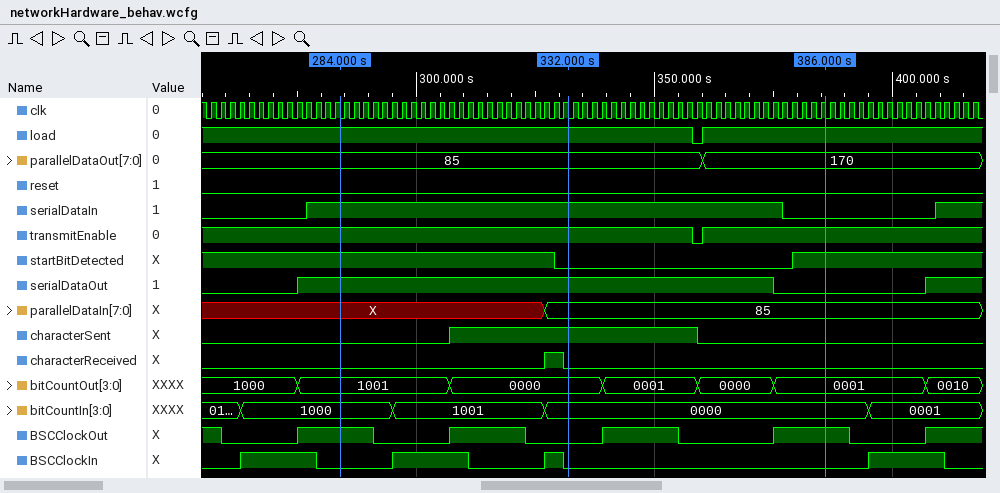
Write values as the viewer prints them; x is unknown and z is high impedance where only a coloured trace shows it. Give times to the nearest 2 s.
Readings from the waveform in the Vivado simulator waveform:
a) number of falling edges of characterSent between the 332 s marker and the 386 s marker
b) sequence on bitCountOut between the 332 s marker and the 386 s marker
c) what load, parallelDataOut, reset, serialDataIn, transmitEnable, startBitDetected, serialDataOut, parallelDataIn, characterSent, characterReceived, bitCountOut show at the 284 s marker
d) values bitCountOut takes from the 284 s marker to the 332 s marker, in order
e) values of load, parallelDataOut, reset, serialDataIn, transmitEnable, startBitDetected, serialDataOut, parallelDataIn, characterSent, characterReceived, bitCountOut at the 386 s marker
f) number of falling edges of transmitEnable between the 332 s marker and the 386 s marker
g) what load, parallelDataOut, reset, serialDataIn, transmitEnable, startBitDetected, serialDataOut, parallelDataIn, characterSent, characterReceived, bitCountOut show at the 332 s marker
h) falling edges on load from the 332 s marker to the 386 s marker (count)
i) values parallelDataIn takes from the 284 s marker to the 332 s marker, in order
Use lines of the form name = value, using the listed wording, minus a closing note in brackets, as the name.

number of falling edges of characterSent between the 332 s marker and the 386 s marker = 1
sequence on bitCountOut between the 332 s marker and the 386 s marker = 0000, 0001, 0000, 0001
what load, parallelDataOut, reset, serialDataIn, transmitEnable, startBitDetected, serialDataOut, parallelDataIn, characterSent, characterReceived, bitCountOut show at the 284 s marker = load=1, parallelDataOut=85, reset=0, serialDataIn=1, transmitEnable=1, startBitDetected=1, serialDataOut=1, parallelDataIn=X, characterSent=0, characterReceived=0, bitCountOut=1001
values bitCountOut takes from the 284 s marker to the 332 s marker, in order = 1001, 0000
values of load, parallelDataOut, reset, serialDataIn, transmitEnable, startBitDetected, serialDataOut, parallelDataIn, characterSent, characterReceived, bitCountOut at the 386 s marker = load=1, parallelDataOut=170, reset=0, serialDataIn=0, transmitEnable=1, startBitDetected=1, serialDataOut=0, parallelDataIn=85, characterSent=0, characterReceived=0, bitCountOut=0001
number of falling edges of transmitEnable between the 332 s marker and the 386 s marker = 1
what load, parallelDataOut, reset, serialDataIn, transmitEnable, startBitDetected, serialDataOut, parallelDataIn, characterSent, characterReceived, bitCountOut show at the 332 s marker = load=1, parallelDataOut=85, reset=0, serialDataIn=1, transmitEnable=1, startBitDetected=0, serialDataOut=1, parallelDataIn=85, characterSent=1, characterReceived=0, bitCountOut=0000
falling edges on load from the 332 s marker to the 386 s marker = 1
values parallelDataIn takes from the 284 s marker to the 332 s marker, in order = X, 85
